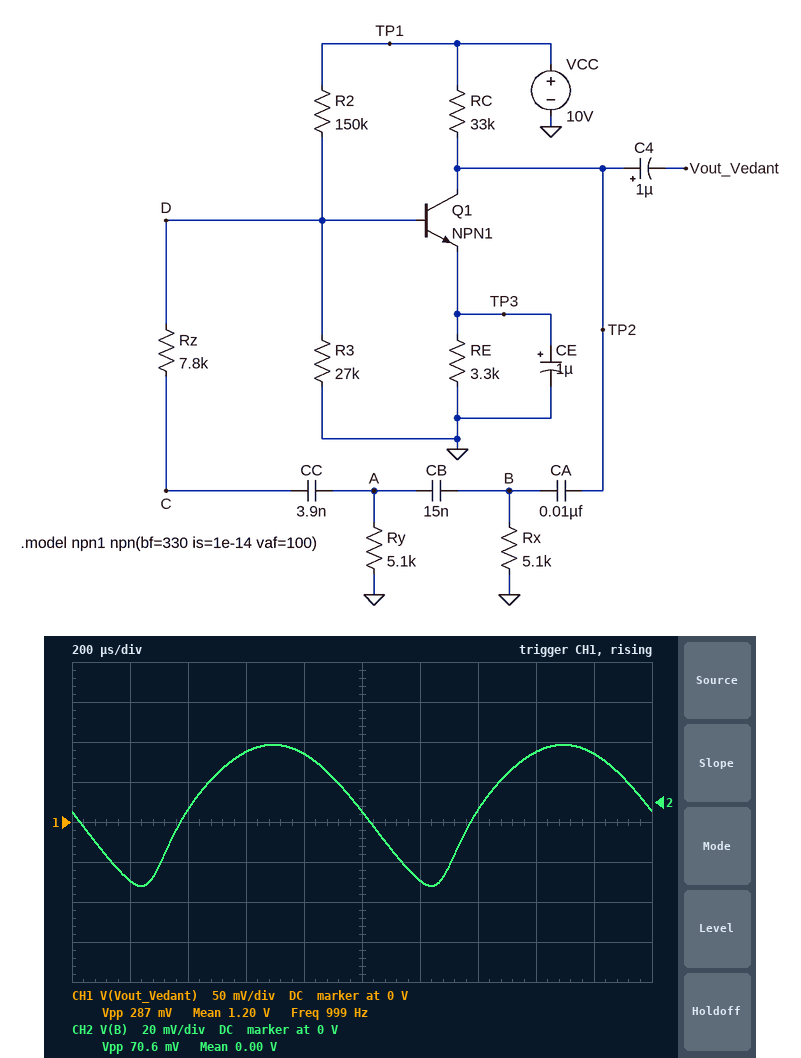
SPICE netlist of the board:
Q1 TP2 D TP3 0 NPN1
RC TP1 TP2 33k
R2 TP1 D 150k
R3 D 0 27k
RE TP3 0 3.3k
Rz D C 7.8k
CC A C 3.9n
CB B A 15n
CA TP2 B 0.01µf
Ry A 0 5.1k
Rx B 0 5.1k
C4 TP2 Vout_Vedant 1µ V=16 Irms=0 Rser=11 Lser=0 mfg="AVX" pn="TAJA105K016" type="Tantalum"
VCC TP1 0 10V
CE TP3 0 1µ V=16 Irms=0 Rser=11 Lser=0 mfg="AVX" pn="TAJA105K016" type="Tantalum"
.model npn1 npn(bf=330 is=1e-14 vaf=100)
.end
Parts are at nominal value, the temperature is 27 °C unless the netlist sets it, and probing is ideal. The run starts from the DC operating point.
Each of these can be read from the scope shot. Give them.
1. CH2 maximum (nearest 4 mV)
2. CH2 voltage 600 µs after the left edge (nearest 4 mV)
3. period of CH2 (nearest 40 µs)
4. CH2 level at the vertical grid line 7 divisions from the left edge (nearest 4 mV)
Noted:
28 mV
24 mV
1.00 ms
-4 mV
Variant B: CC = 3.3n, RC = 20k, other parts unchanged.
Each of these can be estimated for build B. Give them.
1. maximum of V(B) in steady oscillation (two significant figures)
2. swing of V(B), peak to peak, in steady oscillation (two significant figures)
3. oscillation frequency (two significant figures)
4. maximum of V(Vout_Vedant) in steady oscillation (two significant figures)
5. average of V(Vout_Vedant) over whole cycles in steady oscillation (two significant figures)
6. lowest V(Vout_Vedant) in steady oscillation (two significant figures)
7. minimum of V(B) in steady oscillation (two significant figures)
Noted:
780 mV
1.8 V
960 Hz
8.0 V
4.7 V
990 mV
-1.0 V
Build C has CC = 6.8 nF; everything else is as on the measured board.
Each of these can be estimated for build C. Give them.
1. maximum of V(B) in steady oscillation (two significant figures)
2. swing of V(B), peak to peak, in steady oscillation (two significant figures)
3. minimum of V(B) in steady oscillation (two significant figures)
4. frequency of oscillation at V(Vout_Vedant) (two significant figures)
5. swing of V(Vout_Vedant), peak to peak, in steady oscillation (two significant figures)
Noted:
27 mV
66 mV
-40 mV
840 Hz
300 mV
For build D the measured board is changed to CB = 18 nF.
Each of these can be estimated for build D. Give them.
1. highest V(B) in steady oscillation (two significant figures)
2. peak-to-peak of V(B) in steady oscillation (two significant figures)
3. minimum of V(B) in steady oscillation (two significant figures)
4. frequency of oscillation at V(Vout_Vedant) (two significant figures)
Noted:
25 mV
62 mV
-37 mV
940 Hz
